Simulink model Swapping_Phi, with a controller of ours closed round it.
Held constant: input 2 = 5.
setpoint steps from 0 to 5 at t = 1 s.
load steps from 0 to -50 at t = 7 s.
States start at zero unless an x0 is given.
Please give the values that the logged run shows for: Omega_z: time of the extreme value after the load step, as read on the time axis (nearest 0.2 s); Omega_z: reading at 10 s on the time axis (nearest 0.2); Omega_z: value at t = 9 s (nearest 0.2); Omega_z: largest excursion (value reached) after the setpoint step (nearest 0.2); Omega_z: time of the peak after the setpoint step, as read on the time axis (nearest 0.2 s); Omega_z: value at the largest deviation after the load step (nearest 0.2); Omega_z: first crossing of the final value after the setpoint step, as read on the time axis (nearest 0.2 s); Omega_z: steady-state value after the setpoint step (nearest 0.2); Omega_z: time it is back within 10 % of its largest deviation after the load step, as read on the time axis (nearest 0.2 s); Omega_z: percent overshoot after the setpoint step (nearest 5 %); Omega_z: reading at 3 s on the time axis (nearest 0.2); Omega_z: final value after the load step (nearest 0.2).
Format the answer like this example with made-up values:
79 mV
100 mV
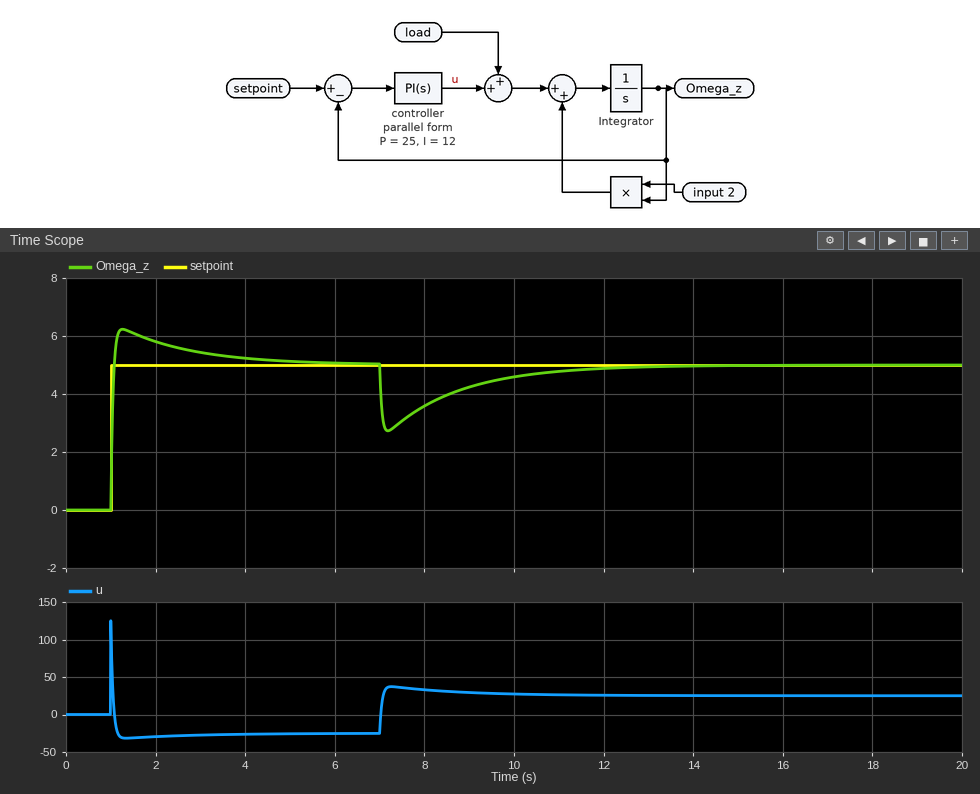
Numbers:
7.2 s
4.6
4.2
6.2
1.2 s
2.8
1.0 s
5.0
11.0 s
25 %
5.4
5.0
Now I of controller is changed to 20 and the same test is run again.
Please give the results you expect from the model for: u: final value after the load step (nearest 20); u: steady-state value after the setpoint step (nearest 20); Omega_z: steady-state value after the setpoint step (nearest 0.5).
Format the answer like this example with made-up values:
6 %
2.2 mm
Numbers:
20
-20
5.0
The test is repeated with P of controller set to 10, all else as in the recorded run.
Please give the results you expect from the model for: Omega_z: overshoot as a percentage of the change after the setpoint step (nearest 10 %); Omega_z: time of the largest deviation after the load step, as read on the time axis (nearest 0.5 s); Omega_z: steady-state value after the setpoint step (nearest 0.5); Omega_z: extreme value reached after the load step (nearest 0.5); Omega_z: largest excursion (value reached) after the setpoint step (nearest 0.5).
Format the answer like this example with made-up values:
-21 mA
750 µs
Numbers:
70 %
7.5 s
5.0
-1.5
8.5
